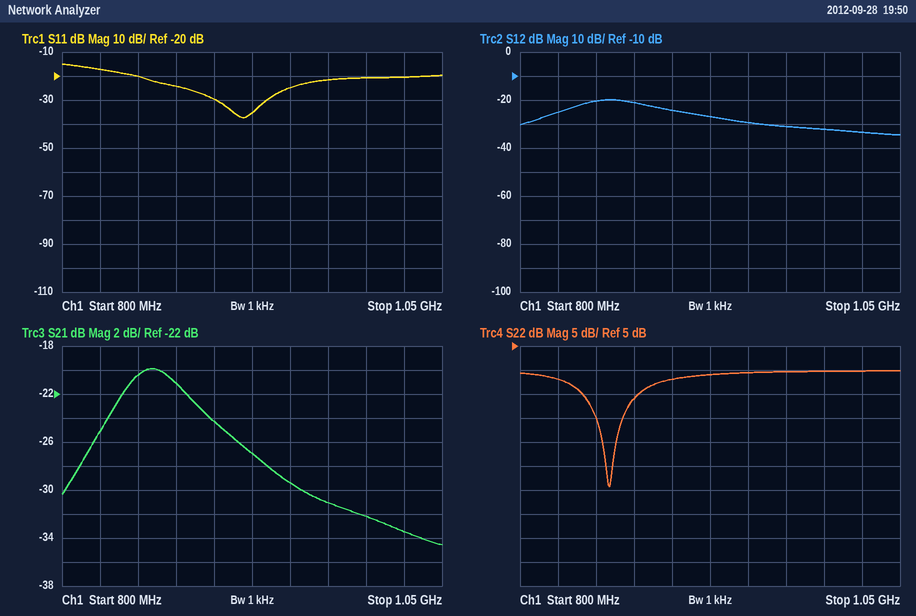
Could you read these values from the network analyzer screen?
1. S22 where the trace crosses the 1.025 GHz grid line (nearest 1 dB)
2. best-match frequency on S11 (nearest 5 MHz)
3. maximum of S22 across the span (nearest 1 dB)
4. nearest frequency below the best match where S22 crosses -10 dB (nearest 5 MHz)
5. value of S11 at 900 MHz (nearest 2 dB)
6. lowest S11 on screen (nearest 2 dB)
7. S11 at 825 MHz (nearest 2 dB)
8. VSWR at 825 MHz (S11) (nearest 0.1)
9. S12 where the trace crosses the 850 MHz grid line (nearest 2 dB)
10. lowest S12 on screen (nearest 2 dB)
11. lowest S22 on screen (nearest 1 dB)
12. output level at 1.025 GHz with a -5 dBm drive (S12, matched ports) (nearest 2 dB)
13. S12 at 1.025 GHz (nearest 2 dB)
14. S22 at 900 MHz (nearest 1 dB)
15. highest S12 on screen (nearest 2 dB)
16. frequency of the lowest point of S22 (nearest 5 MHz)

0 dB
920 MHz
0 dB
850 MHz
-30 dB
-38 dB
-18 dB
1.3
-20 dB
-34 dB
-24 dB
-38 dBm
-34 dB
-2 dB
-20 dB
860 MHz
